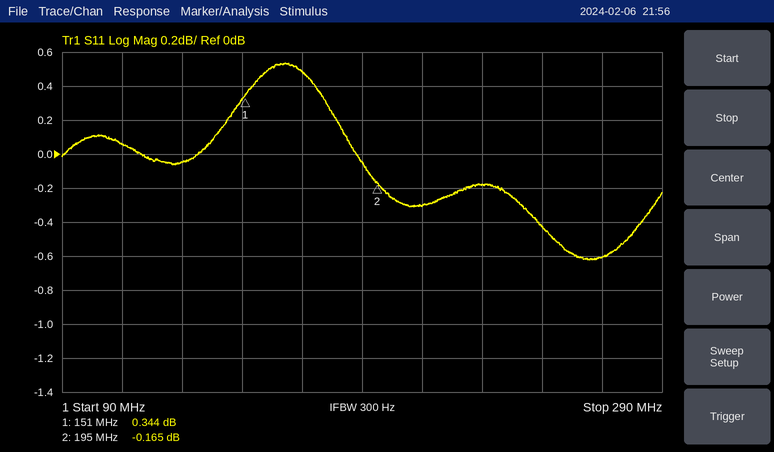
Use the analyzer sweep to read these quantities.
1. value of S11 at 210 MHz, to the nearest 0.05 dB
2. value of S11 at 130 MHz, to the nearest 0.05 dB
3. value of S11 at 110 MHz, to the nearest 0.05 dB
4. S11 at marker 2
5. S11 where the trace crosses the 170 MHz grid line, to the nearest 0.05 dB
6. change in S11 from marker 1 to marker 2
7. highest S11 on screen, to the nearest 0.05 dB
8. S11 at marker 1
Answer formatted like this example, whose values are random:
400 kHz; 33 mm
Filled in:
-0.30 dB; -0.05 dB; 0.05 dB; -0.165 dB; 0.50 dB; -0.509 dB; 0.55 dB; 0.344 dB
